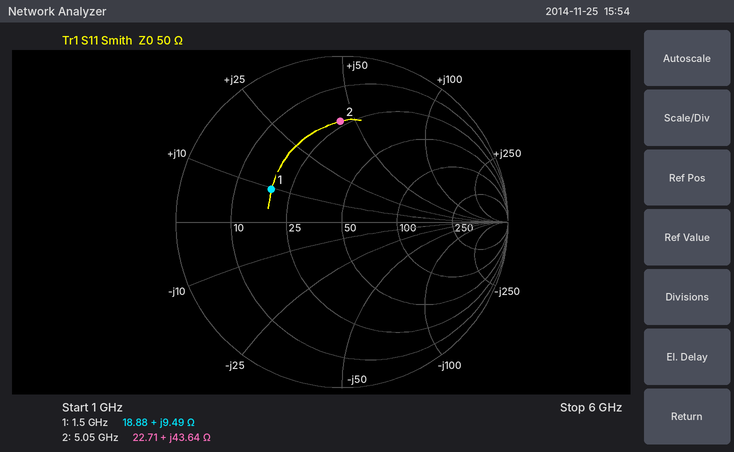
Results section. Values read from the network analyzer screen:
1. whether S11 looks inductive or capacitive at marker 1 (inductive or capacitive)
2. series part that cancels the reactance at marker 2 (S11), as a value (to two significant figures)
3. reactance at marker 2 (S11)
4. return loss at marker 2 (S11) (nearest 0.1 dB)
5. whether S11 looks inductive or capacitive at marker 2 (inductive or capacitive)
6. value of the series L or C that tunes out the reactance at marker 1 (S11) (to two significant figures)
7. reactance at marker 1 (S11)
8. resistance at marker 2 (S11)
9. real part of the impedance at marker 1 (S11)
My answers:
inductive
720 fF
+43.64 Ω
4.3 dB
inductive
11 pF
+9.49 Ω
22.71 Ω
18.88 Ω
